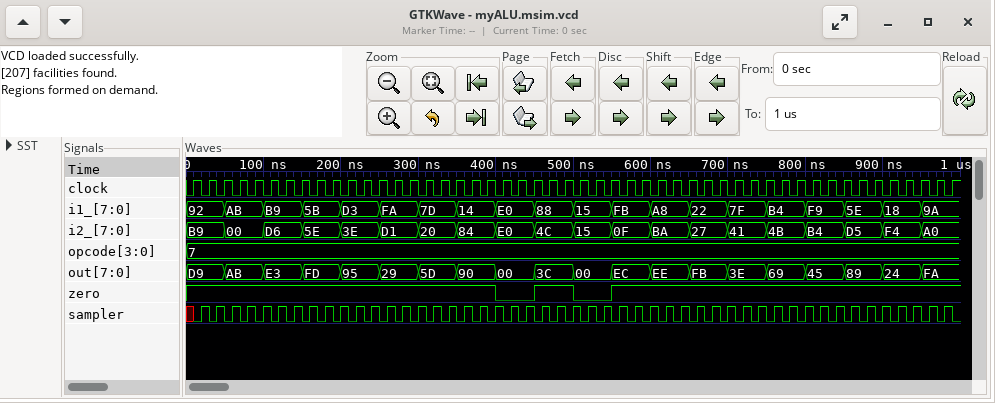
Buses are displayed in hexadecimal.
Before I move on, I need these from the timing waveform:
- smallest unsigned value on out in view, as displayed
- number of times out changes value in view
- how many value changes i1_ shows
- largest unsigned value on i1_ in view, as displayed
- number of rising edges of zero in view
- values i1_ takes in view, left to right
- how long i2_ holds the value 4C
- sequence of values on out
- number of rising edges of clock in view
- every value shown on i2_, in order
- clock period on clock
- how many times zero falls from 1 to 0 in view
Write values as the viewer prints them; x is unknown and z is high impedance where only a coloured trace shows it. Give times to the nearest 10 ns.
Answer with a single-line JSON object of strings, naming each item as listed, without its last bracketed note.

{"smallest unsigned value on out in view, as displayed": "00", "number of times out changes value in view": "19", "how many value changes i1_ shows": "19", "largest unsigned value on i1_ in view, as displayed": "FB", "number of rising edges of zero in view": "2", "values i1_ takes in view, left to right": "92, AB, B9, 5B, D3, FA, 7D, 14, E0, 88, 15, FB, A8, 22, 7F, B4, F9, 5E, 18, 9A", "how long i2_ holds the value 4C": "50 ns", "sequence of values on out": "D9, AB, E3, FD, 95, 29, 5D, 90, 00, 3C, 00, EC, EE, FB, 3E, 69, 45, 89, 24, FA", "number of rising edges of clock in view": "50", "every value shown on i2_, in order": "B9, 00, D6, 5E, 3E, D1, 20, 84, E0, 4C, 15, 0F, BA, 27, 41, 4B, B4, D5, F4, A0", "clock period on clock": "20 ns", "how many times zero falls from 1 to 0 in view": "2"}
